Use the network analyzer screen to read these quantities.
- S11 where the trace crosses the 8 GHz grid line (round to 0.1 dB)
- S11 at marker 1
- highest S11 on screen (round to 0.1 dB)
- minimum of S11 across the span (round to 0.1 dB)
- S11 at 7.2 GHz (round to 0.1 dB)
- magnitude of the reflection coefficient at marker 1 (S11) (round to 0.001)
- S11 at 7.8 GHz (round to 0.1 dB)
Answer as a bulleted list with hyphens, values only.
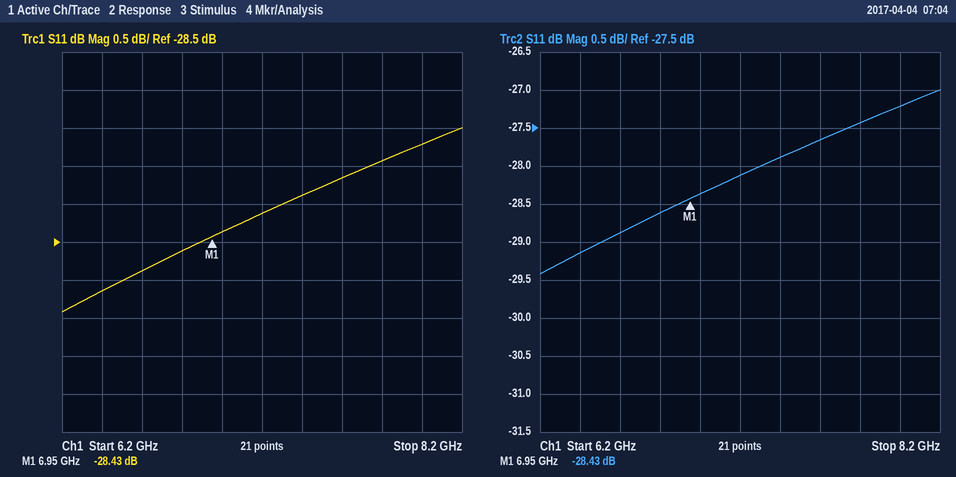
- -27.2 dB
- -28.43 dB
- -27.0 dB
- -29.4 dB
- -28.1 dB
- 0.038
- -27.4 dB
